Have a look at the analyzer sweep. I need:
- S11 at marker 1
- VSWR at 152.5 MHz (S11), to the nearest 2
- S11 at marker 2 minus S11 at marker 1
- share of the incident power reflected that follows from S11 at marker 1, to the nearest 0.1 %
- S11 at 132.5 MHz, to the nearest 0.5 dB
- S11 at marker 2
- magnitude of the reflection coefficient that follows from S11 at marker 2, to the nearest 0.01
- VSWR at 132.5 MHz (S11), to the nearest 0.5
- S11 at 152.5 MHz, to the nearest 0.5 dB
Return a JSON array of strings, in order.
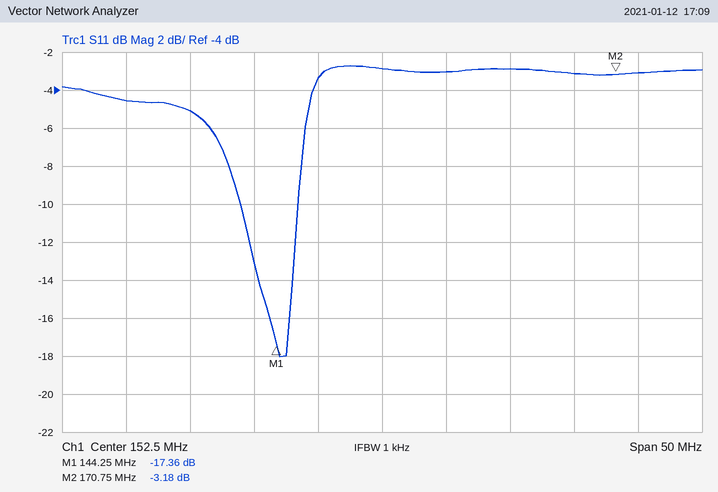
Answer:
["-17.36 dB", "6", "14.18 dB", "1.8 %", "-4.5 dB", "-3.18 dB", "0.69", "4.0", "-3.0 dB"]
